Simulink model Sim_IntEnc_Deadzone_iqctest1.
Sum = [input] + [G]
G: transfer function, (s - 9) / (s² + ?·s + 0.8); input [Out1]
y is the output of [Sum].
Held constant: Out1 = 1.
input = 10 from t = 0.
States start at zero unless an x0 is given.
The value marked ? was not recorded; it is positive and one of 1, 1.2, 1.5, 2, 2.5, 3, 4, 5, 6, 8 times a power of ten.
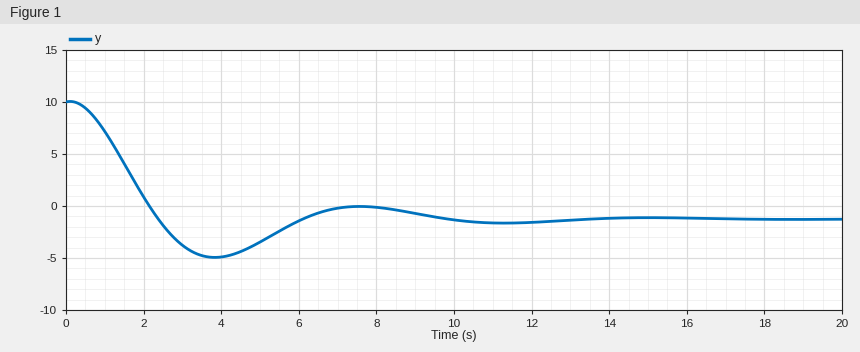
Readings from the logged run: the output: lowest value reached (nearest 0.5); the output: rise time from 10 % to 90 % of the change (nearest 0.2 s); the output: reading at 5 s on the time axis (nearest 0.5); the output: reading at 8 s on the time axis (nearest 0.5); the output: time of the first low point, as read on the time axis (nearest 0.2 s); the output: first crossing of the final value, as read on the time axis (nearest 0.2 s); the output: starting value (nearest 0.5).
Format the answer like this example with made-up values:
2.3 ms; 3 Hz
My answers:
-5.0; 1.6 s; -3.5; 0.0; 3.8 s; 2.4 s; 10.0
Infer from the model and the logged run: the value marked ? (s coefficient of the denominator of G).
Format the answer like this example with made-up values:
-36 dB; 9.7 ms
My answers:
0.6
